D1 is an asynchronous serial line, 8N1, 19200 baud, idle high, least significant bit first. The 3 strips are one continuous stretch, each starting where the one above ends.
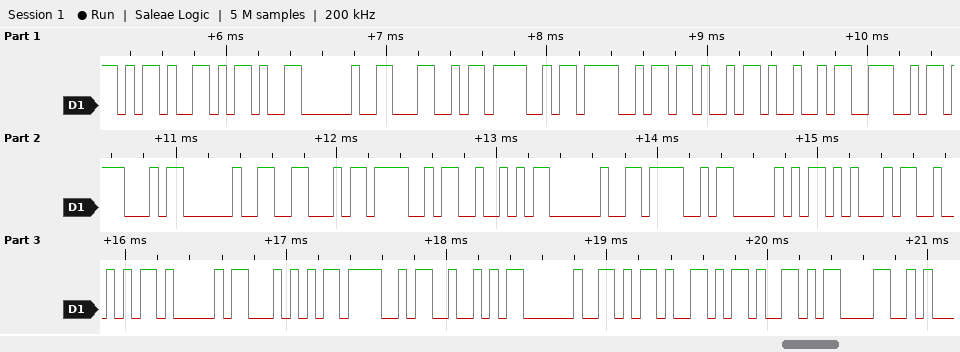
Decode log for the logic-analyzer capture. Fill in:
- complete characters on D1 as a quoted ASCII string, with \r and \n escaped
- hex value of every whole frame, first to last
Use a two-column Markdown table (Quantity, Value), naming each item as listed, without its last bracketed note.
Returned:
| Quantity | Value |
|---|---|
| complete characters on D1 as a quoted ASCII string, with \r and \n escaped | "-- LOOKING FOR OPERATOR --\r" |
| hex value of every whole frame, first to last | 0x2D 0x2D 0x20 0x4C 0x4F 0x4F 0x4B 0x49 0x4E 0x47 0x20 0x46 0x4F 0x52 0x20 0x4F 0x50 0x45 0x52 0x41 0x54 0x4F 0x52 0x20 0x2D 0x2D 0x0D |
